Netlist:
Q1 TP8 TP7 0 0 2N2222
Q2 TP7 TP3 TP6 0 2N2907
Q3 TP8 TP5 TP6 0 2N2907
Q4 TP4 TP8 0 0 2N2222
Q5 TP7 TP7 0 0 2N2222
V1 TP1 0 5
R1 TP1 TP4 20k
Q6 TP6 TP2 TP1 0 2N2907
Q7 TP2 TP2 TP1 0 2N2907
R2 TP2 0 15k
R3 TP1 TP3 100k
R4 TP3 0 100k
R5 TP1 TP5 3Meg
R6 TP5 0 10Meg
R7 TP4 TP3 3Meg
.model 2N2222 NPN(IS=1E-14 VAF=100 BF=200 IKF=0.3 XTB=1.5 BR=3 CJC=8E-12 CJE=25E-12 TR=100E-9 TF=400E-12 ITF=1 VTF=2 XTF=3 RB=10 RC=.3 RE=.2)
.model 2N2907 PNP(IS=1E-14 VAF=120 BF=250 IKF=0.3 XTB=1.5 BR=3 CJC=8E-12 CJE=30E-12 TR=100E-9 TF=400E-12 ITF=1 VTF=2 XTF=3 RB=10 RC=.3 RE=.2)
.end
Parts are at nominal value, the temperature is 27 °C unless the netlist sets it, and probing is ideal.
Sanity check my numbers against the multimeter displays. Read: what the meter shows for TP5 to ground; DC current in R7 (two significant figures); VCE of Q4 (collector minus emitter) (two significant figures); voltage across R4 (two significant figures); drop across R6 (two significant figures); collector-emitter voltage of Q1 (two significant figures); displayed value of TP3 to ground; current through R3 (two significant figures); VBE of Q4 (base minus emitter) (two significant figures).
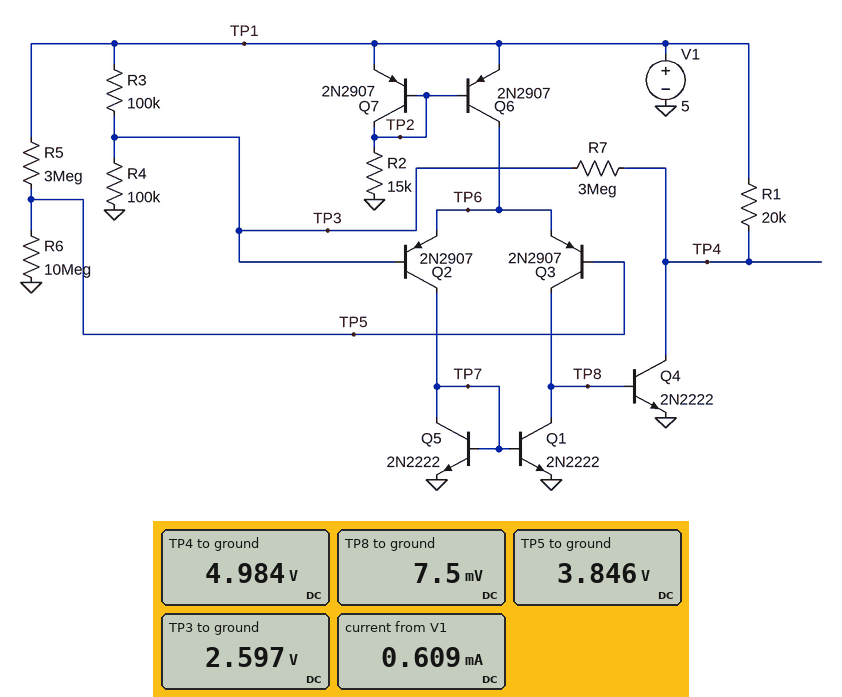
3.846 V
800 nA
5.0 V
2.6 V
3.8 V
7.5 mV
2.597 V
24 µA
7.5 mV
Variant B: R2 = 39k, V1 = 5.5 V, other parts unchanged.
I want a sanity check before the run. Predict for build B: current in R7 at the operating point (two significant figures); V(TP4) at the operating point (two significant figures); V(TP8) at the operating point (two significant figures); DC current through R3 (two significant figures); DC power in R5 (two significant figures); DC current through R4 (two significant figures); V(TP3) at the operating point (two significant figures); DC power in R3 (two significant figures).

890 nA
5.5 V
7.5 mV
27 µA
540 nW
28 µA
2.8 V
72 µW
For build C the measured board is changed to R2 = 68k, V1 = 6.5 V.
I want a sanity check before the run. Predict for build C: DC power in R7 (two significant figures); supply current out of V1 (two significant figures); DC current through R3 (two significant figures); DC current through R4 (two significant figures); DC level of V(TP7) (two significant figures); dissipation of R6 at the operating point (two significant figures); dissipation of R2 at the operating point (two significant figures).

3.3 µW
210 µA
32 µA
33 µA
590 mV
2.5 µW
510 µW
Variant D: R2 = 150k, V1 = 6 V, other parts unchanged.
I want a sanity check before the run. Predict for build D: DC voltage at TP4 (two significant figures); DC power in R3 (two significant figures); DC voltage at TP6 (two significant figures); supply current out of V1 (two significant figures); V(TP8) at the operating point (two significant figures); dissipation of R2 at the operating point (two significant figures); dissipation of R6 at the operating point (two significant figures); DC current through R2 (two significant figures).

6.0 V
87 µW
3.6 V
100 µA
7.5 mV
200 µW
2.1 µW
36 µA
